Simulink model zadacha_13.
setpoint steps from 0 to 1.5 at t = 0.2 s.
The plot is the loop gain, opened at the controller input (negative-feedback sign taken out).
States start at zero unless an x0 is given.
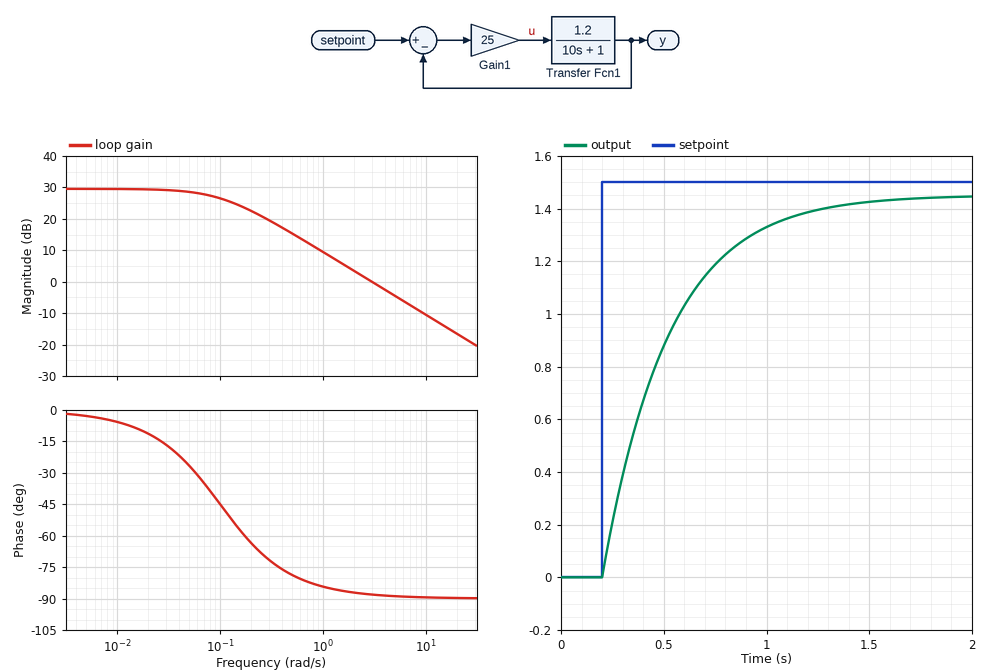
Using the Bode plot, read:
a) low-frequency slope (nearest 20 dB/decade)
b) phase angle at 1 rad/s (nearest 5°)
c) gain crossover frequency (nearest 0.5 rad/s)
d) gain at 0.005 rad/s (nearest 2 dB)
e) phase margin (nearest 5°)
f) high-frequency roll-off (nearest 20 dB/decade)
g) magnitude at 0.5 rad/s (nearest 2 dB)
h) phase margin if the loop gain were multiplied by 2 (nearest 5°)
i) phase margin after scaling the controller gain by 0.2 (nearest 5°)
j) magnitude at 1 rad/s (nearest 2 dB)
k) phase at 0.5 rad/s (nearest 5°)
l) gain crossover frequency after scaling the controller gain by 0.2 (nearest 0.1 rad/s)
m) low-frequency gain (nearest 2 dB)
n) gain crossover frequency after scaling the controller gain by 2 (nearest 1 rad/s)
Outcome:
0 dB/decade
-85°
3.0 rad/s
30 dB
90°
-20 dB/decade
16 dB
90°
100°
10 dB
-80°
0.6 rad/s
30 dB
6 rad/s
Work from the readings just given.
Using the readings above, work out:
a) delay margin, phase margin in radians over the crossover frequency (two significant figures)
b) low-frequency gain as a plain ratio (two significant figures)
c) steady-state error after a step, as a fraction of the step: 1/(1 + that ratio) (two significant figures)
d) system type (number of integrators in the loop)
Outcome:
0.52 s
32
0.030
0
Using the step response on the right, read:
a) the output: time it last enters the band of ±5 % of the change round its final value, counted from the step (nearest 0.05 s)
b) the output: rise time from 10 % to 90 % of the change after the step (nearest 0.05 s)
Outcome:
0.95 s
0.70 s
